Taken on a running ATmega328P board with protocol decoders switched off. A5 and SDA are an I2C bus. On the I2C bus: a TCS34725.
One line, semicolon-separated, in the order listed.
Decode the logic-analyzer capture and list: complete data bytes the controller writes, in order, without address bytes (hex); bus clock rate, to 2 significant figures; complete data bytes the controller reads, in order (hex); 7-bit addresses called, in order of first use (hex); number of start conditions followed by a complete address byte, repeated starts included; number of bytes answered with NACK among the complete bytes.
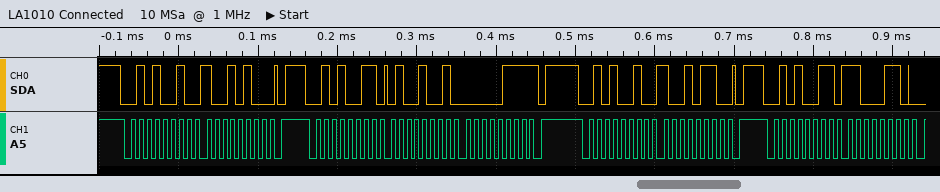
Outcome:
94 96; 100 kHz; 49 07 C6; 0x29; 4; 1
